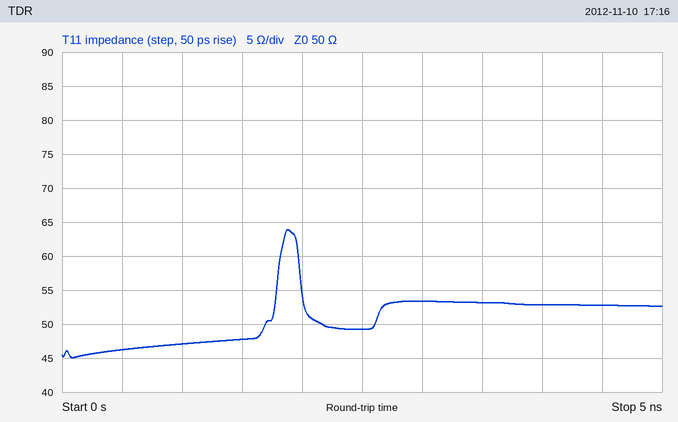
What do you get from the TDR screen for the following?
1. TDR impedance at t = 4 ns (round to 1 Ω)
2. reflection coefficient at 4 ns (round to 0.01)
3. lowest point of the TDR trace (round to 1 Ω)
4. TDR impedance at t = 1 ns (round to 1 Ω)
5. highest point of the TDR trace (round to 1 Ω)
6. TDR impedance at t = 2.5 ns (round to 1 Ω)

53 Ω
+0.03
45 Ω
47 Ω
64 Ω
49 Ω
